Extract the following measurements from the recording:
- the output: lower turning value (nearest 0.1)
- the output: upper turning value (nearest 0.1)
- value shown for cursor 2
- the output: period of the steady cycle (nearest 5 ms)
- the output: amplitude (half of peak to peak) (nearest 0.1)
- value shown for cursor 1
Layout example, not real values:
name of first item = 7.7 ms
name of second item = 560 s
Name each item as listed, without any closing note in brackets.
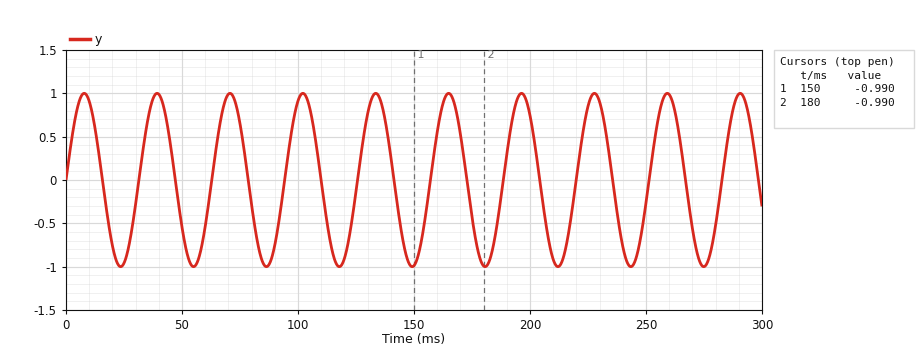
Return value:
the output: lower turning value = -1.0
the output: upper turning value = 1.0
value shown for cursor 2 = -0.990
the output: period of the steady cycle = 30 ms
the output: amplitude (half of peak to peak) = 1.0
value shown for cursor 1 = -0.990
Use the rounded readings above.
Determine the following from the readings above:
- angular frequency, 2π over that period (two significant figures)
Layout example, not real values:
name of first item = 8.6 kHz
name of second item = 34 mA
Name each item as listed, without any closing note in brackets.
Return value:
angular frequency, 2π over that period = 0.21 rad/ms
